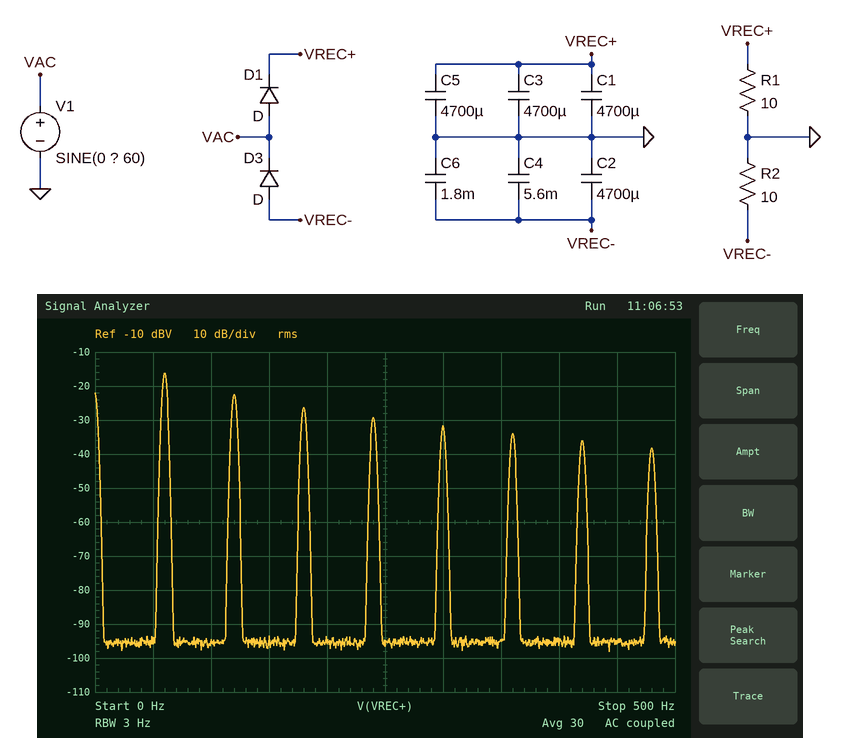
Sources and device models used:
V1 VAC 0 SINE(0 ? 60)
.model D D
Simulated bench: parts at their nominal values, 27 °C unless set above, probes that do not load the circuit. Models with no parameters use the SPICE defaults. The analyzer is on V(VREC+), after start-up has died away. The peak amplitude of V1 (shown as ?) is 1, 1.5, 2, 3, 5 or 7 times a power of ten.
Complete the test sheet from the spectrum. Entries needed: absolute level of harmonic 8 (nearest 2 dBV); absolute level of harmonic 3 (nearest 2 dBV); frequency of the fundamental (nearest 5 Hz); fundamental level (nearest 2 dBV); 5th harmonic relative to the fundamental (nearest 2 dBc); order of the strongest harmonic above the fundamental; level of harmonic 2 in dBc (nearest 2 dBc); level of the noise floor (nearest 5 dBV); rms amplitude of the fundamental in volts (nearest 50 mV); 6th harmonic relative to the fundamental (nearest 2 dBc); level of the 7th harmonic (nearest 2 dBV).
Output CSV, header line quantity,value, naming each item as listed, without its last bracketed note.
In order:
quantity,value
absolute level of harmonic 8,-38 dBV
absolute level of harmonic 3,-26 dBV
frequency of the fundamental,60 Hz
fundamental level,-16 dBV
5th harmonic relative to the fundamental,-16 dBc
order of the strongest harmonic above the fundamental,2
level of harmonic 2 in dBc,-6 dBc
level of the noise floor,-95 dBV
rms amplitude of the fundamental in volts,150 mV
6th harmonic relative to the fundamental,-18 dBc
level of the 7th harmonic,-36 dBV
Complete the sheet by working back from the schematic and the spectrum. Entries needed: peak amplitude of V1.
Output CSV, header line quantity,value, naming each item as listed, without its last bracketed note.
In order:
quantity,value
peak amplitude of V1,7 V
